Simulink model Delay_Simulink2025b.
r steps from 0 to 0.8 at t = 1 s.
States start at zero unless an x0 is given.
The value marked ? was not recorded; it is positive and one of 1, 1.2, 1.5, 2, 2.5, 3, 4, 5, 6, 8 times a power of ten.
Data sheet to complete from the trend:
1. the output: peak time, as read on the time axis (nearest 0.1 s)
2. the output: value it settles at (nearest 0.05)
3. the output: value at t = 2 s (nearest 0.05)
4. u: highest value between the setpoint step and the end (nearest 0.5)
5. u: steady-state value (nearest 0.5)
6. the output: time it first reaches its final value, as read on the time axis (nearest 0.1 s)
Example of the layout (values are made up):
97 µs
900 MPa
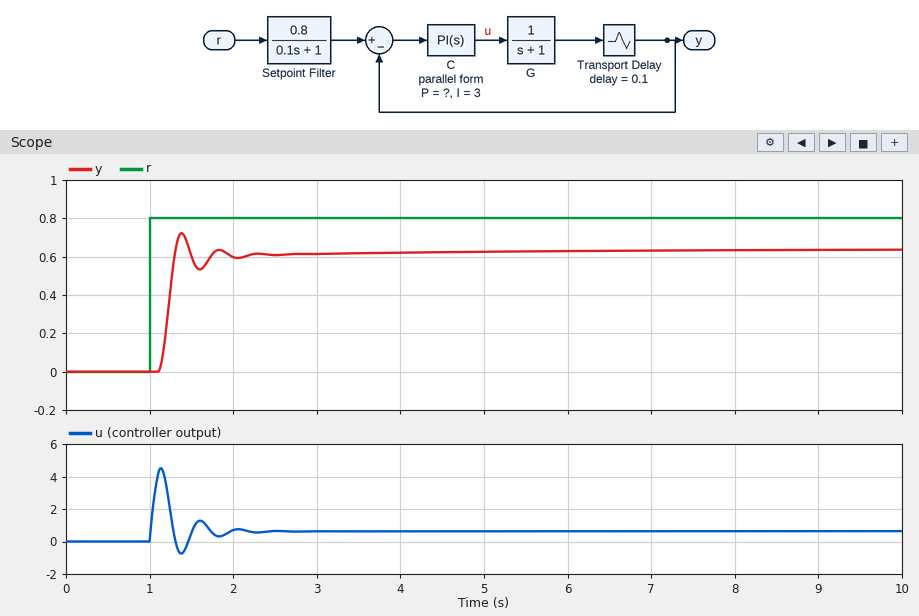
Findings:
1.4 s
0.65
0.60
4.5
0.5
1.3 s
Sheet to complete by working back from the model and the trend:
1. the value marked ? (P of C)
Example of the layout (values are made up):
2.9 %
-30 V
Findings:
10
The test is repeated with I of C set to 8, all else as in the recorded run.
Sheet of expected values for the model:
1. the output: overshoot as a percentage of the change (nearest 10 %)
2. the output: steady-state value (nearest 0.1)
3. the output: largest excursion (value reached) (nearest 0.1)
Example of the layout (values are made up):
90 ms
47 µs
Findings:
20 %
0.6
0.8
